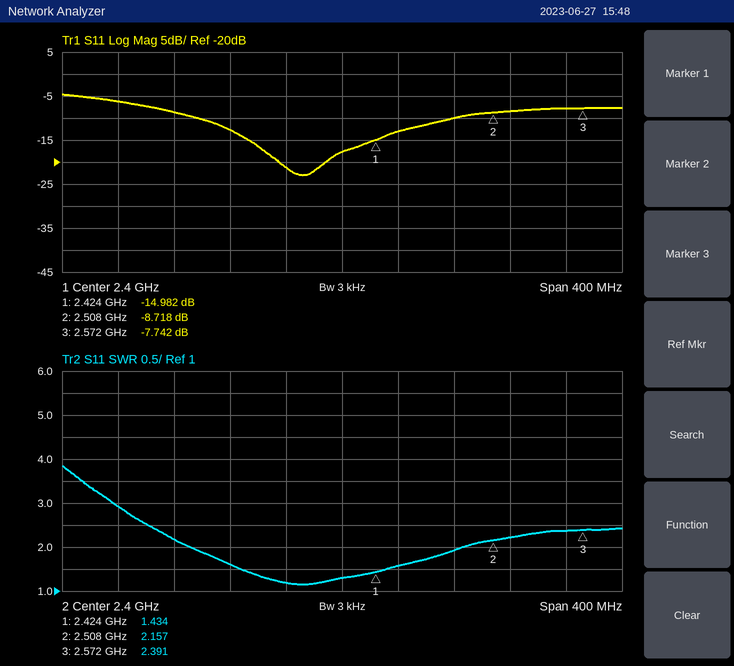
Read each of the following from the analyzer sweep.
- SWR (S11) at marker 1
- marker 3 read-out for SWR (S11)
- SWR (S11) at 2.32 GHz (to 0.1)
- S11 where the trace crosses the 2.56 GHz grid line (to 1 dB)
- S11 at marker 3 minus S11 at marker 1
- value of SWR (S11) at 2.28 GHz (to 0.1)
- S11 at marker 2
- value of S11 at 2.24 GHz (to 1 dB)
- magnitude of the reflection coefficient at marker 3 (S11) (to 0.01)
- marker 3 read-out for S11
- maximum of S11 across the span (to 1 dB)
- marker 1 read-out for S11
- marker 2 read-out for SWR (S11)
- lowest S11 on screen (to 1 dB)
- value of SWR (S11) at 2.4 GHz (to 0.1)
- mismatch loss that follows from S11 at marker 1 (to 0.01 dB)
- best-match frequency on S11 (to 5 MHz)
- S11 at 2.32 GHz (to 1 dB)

1.434
2.391
1.6
-8 dB
7.240 dB
2.2
-8.718 dB
-6 dB
0.41
-7.742 dB
-5 dB
-14.982 dB
2.157
-23 dB
1.3
0.14 dB
2.370 GHz
-13 dB
